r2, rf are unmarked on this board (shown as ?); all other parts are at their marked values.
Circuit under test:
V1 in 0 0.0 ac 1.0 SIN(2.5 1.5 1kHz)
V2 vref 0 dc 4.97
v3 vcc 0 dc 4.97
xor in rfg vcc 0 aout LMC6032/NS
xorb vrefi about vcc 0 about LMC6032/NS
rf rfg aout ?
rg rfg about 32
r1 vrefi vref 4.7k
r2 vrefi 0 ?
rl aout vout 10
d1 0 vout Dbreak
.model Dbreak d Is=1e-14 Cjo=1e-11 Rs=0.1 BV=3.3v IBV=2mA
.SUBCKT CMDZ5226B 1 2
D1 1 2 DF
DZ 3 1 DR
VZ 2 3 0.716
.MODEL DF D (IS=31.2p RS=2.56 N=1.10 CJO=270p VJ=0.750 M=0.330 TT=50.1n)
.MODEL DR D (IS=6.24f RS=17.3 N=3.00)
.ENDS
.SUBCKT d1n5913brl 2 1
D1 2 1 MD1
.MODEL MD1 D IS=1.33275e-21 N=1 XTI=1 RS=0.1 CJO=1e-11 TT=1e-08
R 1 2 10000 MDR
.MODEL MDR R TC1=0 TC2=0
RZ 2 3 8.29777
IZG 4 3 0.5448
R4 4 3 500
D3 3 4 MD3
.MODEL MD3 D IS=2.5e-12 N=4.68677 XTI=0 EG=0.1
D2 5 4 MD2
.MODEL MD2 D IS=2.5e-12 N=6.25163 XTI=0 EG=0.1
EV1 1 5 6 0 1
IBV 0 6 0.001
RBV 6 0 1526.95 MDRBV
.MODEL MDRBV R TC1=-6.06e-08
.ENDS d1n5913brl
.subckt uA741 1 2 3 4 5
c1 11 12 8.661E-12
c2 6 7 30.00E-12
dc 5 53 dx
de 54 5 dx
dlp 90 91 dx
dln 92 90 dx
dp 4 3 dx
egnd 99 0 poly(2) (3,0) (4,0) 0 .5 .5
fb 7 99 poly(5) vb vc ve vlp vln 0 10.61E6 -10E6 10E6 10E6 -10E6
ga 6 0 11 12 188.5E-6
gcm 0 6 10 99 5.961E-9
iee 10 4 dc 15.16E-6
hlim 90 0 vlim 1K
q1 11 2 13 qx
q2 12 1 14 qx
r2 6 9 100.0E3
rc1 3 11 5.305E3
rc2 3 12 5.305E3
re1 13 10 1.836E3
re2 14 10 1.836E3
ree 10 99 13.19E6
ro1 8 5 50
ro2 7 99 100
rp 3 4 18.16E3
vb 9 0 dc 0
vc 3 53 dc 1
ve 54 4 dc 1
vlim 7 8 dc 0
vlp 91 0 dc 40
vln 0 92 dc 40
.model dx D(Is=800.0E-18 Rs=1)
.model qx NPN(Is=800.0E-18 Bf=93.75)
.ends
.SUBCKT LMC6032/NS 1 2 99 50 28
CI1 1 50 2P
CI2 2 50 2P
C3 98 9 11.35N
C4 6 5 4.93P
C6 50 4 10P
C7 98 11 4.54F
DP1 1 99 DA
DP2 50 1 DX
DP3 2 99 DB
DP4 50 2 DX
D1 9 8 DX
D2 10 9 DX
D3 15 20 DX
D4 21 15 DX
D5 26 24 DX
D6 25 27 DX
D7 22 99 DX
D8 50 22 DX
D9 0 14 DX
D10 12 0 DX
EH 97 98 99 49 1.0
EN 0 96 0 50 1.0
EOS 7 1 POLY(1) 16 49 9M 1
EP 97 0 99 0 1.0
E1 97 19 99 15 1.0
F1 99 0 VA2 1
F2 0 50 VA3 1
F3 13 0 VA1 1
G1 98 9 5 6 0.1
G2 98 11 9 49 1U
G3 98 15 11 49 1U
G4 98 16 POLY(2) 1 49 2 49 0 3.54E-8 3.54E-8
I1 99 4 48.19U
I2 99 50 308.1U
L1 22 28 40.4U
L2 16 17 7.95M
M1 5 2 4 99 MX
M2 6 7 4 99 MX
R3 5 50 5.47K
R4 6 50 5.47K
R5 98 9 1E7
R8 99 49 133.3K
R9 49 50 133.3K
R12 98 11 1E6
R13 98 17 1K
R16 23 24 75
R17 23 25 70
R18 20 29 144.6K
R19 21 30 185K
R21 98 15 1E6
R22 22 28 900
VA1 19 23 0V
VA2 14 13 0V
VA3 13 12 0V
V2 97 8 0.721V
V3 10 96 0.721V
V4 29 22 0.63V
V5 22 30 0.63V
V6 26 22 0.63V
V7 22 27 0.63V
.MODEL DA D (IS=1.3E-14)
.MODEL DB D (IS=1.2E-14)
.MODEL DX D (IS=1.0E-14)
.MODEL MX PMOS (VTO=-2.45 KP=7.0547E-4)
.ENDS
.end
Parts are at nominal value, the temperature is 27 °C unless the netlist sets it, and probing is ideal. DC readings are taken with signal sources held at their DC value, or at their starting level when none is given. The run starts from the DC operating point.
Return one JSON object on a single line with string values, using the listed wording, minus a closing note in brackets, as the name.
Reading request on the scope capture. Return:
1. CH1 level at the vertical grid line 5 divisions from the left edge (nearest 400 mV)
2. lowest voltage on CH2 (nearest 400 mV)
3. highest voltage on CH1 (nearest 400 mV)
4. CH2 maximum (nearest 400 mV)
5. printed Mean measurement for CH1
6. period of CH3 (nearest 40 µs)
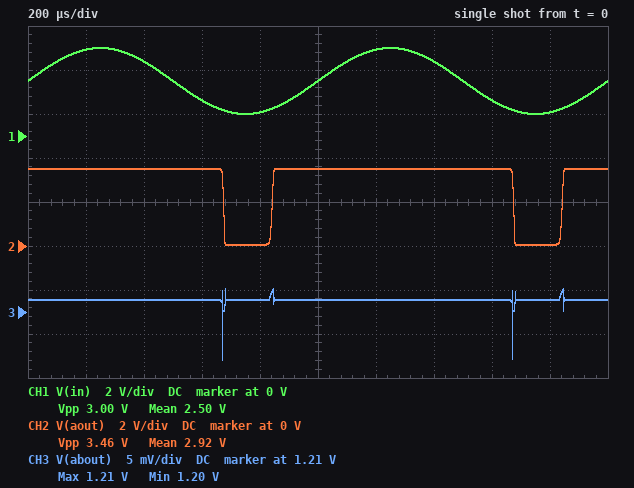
{"CH1 level at the vertical grid line 5 divisions from the left edge": "2.4 V", "lowest voltage on CH2": "0 V", "highest voltage on CH1": "4.0 V", "CH2 maximum": "3.6 V", "printed Mean measurement for CH1": "2.50 V", "period of CH3": "1.00 ms"}
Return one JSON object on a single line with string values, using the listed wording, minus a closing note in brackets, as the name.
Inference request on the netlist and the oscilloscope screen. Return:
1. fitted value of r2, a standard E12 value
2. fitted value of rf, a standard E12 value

{"fitted value of r2, a standard E12 value": "1.5 kΩ", "fitted value of rf, a standard E12 value": "3.3 kΩ"}
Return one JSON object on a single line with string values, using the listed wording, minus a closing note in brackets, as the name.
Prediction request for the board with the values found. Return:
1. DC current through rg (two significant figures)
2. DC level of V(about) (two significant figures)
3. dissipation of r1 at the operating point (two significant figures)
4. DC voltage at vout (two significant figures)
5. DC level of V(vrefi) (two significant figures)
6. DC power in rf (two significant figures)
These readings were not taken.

{"DC current through rg": "360 µA", "DC level of V(about)": "1.2 V", "dissipation of r1 at the operating point": "3.0 mW", "DC voltage at vout": "17 mV", "DC level of V(vrefi)": "1.2 V", "DC power in rf": "420 µW"}
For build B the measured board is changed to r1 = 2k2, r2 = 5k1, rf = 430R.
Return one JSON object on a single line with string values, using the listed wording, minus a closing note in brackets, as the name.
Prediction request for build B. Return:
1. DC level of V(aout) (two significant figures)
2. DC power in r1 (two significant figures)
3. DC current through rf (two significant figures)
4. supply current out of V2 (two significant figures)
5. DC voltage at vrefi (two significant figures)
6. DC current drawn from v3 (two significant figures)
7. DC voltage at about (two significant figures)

{"DC level of V(aout)": "470 mV", "DC power in r1": "1.0 mW", "DC current through rf": "5.6 mA", "supply current out of V2": "680 µA", "DC voltage at vrefi": "3.5 V", "DC current drawn from v3": "6.3 mA", "DC voltage at about": "3.1 V"}
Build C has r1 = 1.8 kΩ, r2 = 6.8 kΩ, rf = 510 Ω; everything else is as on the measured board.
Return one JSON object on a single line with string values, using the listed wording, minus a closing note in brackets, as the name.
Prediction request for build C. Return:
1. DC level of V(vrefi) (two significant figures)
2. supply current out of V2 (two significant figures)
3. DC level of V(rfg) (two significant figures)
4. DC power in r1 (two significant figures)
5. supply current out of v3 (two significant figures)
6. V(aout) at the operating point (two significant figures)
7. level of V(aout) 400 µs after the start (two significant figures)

{"DC level of V(vrefi)": "3.9 V", "supply current out of V2": "580 µA", "DC level of V(rfg)": "2.9 V", "DC power in r1": "600 µW", "supply current out of v3": "5.6 mA", "V(aout) at the operating point": "420 mV", "level of V(aout) 400 µs after the start": "1.3 V"}
